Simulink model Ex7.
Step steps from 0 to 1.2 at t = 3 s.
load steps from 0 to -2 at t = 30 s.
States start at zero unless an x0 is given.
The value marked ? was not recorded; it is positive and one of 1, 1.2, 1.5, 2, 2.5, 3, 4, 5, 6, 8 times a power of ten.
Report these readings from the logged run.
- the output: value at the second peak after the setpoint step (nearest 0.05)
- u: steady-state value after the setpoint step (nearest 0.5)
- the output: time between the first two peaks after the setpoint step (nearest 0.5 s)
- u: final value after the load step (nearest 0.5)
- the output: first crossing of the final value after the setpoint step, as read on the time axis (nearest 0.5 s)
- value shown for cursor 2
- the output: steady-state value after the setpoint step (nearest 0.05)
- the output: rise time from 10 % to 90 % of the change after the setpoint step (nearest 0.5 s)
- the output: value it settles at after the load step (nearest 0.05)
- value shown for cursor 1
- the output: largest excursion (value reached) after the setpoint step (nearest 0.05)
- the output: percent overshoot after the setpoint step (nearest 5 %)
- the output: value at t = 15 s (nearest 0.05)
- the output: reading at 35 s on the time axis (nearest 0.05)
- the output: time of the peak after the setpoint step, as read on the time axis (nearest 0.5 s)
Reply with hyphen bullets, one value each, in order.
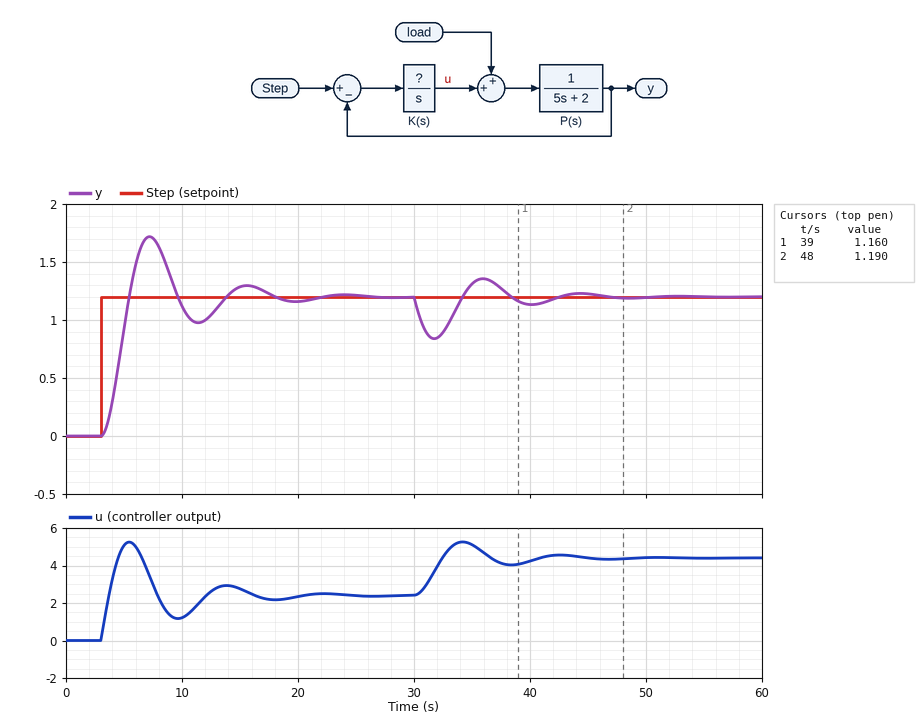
- 1.30
- 2.5
- 8.5 s
- 4.5
- 5.5 s
- 1.190
- 1.20
- 1.5 s
- 1.20
- 1.160
- 1.70
- 45 %
- 1.30
- 1.30
- 7.0 s
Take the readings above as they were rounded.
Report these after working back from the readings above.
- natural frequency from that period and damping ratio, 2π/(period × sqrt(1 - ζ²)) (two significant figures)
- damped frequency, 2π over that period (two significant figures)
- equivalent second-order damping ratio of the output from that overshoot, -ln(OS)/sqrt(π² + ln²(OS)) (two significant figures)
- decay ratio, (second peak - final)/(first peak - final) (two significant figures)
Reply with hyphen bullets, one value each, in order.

- 0.76 rad/s
- 0.74 rad/s
- 0.25
- 0.20
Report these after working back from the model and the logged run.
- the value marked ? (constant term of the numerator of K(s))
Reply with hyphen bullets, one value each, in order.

- 3
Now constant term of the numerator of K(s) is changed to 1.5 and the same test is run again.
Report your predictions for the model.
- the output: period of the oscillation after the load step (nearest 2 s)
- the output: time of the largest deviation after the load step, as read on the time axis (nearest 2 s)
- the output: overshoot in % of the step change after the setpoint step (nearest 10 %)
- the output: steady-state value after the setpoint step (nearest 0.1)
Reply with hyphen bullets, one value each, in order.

- 12 s
- 32 s
- 30 %
- 1.2
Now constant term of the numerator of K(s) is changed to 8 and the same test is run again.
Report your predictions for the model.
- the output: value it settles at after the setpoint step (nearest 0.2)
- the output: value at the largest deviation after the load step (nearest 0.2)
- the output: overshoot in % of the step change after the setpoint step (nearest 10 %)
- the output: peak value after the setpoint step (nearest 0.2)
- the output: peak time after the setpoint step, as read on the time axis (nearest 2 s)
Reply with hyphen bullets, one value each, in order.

- 1.2
- 1.0
- 60 %
- 2.0
- 6 s
